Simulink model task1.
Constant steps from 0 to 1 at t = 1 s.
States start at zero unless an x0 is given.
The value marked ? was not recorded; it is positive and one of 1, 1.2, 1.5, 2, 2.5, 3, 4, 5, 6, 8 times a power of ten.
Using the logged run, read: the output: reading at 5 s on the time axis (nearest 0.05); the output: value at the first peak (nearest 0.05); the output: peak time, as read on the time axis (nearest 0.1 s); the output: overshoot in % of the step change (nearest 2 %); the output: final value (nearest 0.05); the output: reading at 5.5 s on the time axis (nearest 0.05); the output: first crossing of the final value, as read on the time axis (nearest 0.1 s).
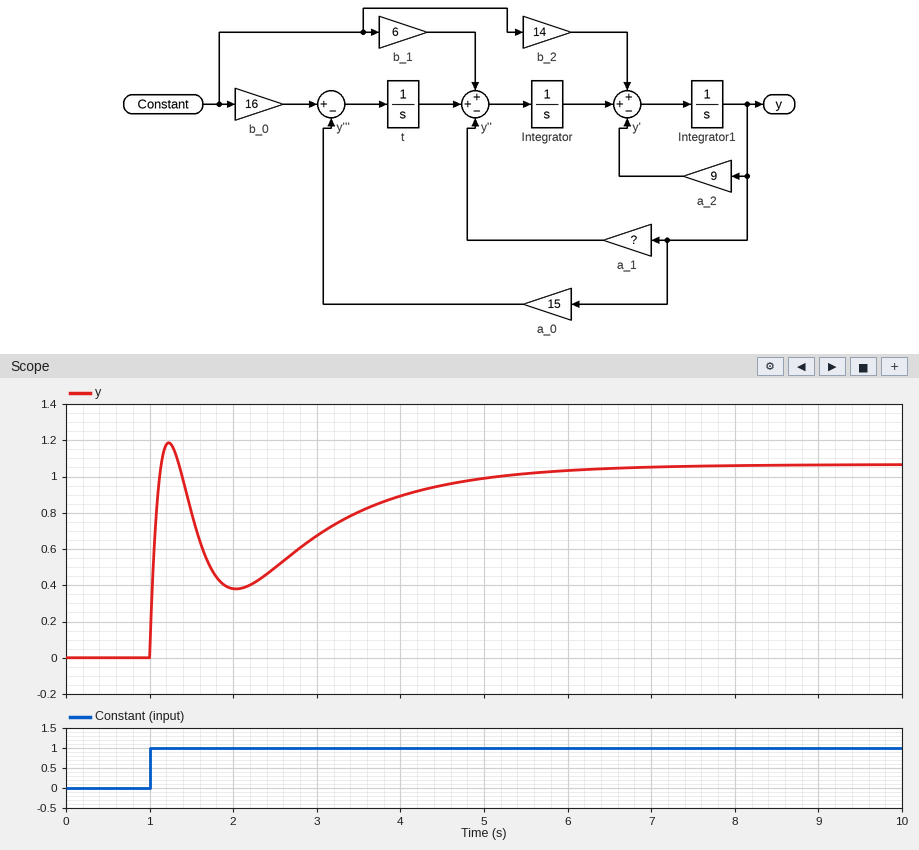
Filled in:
1.00
1.20
1.2 s
12 %
1.05
1.00
1.1 s
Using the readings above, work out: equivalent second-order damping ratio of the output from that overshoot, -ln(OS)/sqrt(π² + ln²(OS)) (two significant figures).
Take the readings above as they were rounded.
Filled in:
0.56
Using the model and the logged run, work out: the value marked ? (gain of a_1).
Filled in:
25
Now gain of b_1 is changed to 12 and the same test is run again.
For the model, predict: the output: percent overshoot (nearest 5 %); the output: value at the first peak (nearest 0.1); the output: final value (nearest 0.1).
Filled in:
20 %
1.3
1.1
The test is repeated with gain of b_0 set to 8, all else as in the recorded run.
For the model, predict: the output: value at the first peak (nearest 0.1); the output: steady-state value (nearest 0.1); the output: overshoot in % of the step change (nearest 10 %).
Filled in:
1.2
0.5
120 %
